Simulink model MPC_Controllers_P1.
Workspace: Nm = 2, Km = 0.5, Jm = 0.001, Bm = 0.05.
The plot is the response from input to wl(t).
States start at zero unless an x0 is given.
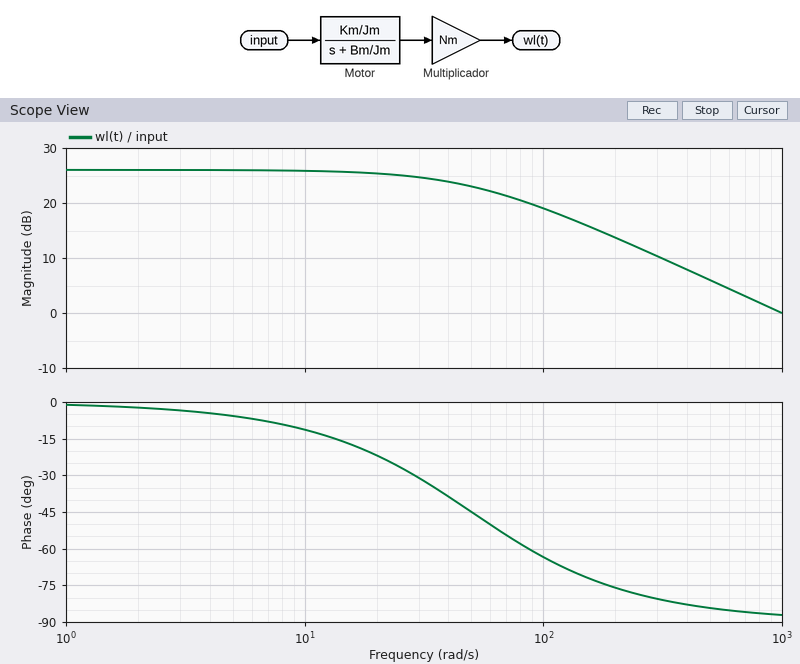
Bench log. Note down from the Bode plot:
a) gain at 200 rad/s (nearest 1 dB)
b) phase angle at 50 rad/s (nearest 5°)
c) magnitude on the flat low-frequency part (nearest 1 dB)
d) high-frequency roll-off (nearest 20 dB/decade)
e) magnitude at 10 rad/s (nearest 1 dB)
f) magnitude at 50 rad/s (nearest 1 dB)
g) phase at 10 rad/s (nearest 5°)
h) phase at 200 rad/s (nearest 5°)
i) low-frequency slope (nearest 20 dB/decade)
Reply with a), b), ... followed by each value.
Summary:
a) 14 dB
b) -45°
c) 26 dB
d) -20 dB/decade
e) 26 dB
f) 23 dB
g) -10°
h) -75°
i) 0 dB/decade
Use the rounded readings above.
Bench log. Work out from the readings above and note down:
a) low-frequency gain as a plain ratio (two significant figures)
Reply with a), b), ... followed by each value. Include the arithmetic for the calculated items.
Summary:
a) 10^(26 / 20) = 20
